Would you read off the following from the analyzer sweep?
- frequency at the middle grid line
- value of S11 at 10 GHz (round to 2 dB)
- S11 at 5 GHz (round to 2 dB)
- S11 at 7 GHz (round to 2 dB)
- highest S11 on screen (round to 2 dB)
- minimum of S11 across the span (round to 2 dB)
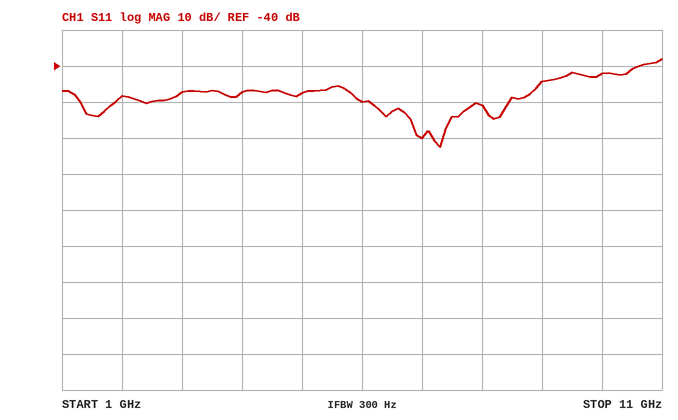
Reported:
6 GHz
-42 dB
-48 dB
-60 dB
-38 dB
-62 dB
